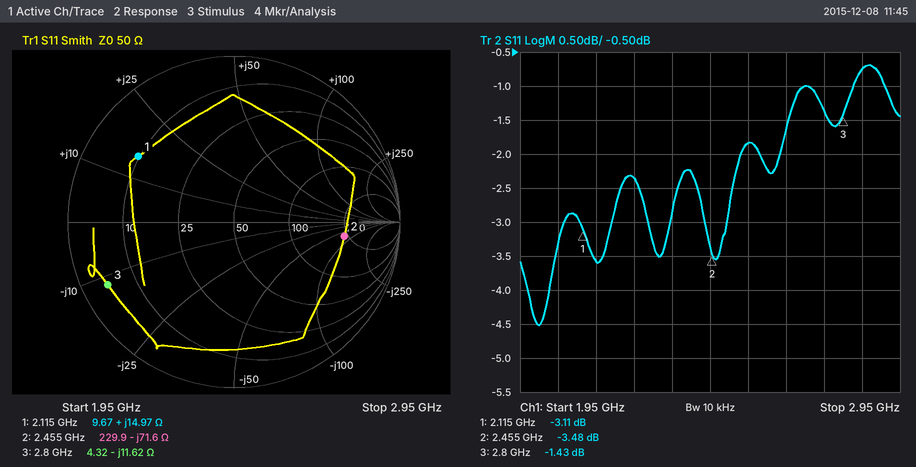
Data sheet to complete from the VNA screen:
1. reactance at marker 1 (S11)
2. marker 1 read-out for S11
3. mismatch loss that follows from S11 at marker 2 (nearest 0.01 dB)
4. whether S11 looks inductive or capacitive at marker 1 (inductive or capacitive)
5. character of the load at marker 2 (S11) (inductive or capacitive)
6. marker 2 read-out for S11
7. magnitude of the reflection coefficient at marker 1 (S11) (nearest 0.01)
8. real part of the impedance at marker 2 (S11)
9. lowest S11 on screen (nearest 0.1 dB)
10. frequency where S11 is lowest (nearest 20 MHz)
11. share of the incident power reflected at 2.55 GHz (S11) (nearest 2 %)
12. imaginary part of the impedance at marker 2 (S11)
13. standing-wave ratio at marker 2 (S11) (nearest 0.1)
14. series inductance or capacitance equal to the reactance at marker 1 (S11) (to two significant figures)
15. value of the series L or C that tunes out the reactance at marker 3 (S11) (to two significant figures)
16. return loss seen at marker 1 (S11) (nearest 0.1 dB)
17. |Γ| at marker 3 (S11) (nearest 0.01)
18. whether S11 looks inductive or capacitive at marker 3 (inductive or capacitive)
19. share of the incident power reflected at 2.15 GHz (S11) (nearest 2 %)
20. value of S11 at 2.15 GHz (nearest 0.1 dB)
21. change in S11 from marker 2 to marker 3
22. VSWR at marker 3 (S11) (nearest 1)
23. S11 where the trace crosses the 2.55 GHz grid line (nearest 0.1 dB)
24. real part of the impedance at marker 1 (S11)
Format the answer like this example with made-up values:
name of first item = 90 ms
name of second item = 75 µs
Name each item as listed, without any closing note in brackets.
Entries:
reactance at marker 1 = +14.97 Ω
marker 1 read-out for S11 = -3.11 dB
mismatch loss that follows from S11 at marker 2 = 2.59 dB
whether S11 looks inductive or capacitive at marker 1 = inductive
character of the load at marker 2 (S11) = capacitive
marker 2 read-out for S11 = -3.48 dB
magnitude of the reflection coefficient at marker 1 (S11) = 0.70
real part of the impedance at marker 2 = 229.9 Ω
lowest S11 on screen = -4.5 dB
frequency where S11 is lowest = 2.00 GHz
share of the incident power reflected at 2.55 GHz (S11) = 66 %
imaginary part of the impedance at marker 2 = -71.6 Ω
standing-wave ratio at marker 2 (S11) = 5.1
series inductance or capacitance equal to the reactance at marker 1 (S11) = 1.1 nH
value of the series L or C that tunes out the reactance at marker 3 (S11) = 660 pH
return loss seen at marker 1 (S11) = 3.1 dB
|Γ| at marker 3 (S11) = 0.85
whether S11 looks inductive or capacitive at marker 3 = capacitive
share of the incident power reflected at 2.15 GHz (S11) = 44 %
value of S11 at 2.15 GHz = -3.6 dB
change in S11 from marker 2 to marker 3 = 2.05 dB
VSWR at marker 3 (S11) = 12
S11 where the trace crosses the 2.55 GHz grid line = -1.8 dB
real part of the impedance at marker 1 = 9.67 Ω
